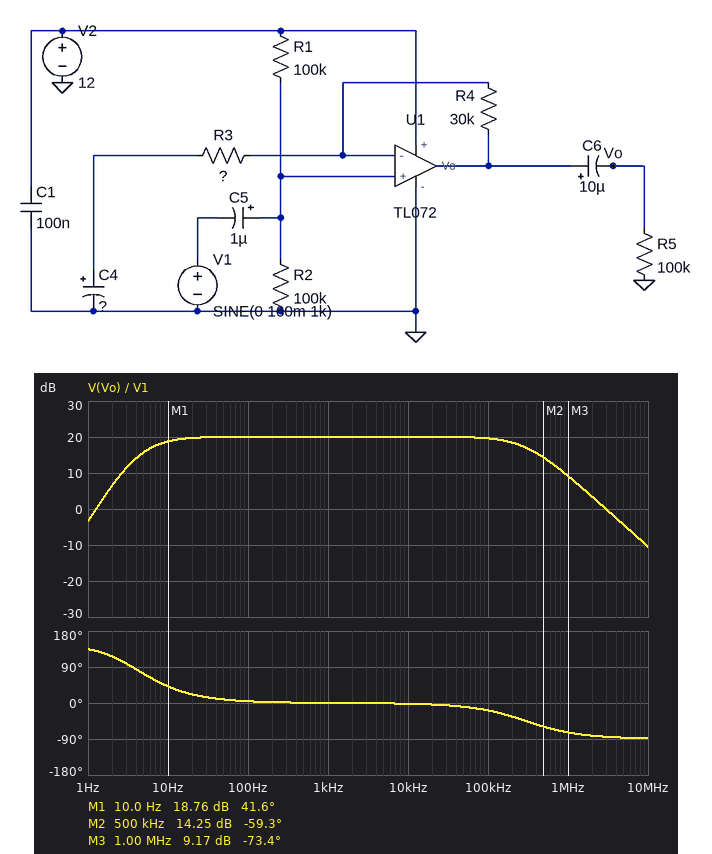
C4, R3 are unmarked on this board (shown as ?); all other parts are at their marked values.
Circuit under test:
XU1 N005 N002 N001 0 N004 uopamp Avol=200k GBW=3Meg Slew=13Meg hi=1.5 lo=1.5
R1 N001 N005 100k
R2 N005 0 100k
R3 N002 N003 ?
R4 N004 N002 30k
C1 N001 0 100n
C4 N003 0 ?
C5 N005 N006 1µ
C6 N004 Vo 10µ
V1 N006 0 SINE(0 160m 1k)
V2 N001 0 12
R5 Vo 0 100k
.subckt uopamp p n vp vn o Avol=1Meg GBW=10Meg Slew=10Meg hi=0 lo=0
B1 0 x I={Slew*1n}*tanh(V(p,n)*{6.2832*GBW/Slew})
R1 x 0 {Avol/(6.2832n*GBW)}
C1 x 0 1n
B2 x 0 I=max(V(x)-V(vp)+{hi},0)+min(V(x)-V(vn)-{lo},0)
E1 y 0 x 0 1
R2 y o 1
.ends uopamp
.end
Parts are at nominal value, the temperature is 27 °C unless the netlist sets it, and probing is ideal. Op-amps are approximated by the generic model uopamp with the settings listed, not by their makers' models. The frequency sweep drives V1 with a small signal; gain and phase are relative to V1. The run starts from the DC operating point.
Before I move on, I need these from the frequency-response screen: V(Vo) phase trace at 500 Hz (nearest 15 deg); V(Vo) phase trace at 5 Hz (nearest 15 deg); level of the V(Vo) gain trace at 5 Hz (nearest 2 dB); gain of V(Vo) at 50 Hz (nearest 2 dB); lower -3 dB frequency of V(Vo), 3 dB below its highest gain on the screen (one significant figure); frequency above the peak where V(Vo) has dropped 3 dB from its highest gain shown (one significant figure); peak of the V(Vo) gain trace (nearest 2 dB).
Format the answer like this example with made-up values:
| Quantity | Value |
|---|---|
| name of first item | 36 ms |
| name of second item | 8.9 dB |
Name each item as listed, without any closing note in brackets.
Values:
| Quantity | Value |
|---|---|
| V(Vo) phase trace at 500 Hz | 0 deg |
| V(Vo) phase trace at 5 Hz | 75 deg |
| level of the V(Vo) gain trace at 5 Hz | 16 dB |
| gain of V(Vo) at 50 Hz | 20 dB |
| lower -3 dB frequency of V(Vo), 3 dB below its highest gain on the screen | 6 Hz |
| frequency above the peak where V(Vo) has dropped 3 dB from its highest gain shown | 300 kHz |
| peak of the V(Vo) gain trace | 20 dB |
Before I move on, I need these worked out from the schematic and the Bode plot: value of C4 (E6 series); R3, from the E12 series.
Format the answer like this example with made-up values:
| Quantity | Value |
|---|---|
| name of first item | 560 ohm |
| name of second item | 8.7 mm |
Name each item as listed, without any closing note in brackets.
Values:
| Quantity | Value |
|---|---|
| value of C4 | 10 µF |
| R3, from the E12 series | 3.3 kΩ |
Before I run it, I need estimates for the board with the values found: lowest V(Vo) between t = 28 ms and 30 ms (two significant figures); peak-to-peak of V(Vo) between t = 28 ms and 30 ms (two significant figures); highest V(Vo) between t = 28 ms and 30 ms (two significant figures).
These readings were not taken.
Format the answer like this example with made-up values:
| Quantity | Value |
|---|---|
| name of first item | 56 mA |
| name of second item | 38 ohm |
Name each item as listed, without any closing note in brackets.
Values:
| Quantity | Value |
|---|---|
| lowest V(Vo) between t = 28 ms and 30 ms | -1.6 V |
| peak-to-peak of V(Vo) between t = 28 ms and 30 ms | 3.2 V |
| highest V(Vo) between t = 28 ms and 30 ms | 1.6 V |
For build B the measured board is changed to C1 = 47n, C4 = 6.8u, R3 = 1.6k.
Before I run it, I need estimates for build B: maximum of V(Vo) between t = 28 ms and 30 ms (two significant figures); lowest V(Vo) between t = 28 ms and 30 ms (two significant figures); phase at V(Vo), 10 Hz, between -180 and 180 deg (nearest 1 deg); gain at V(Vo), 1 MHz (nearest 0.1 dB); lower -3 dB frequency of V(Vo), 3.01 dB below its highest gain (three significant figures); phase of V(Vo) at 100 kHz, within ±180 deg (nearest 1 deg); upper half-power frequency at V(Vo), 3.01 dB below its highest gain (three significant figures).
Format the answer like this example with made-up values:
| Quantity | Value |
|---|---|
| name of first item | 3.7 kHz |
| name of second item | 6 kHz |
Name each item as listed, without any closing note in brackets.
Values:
| Quantity | Value |
|---|---|
| maximum of V(Vo) between t = 28 ms and 30 ms | 3.2 V |
| lowest V(Vo) between t = 28 ms and 30 ms | -3.2 V |
| phase at V(Vo), 10 Hz, between -180 and 180 deg | 70 deg |
| gain at V(Vo), 1 MHz | 9.4 dB |
| lower -3 dB frequency of V(Vo), 3.01 dB below its highest gain | 15.2 Hz |
| phase of V(Vo) at 100 kHz, within ±180 deg | -33 deg |
| upper half-power frequency at V(Vo), 3.01 dB below its highest gain | 152 kHz |
